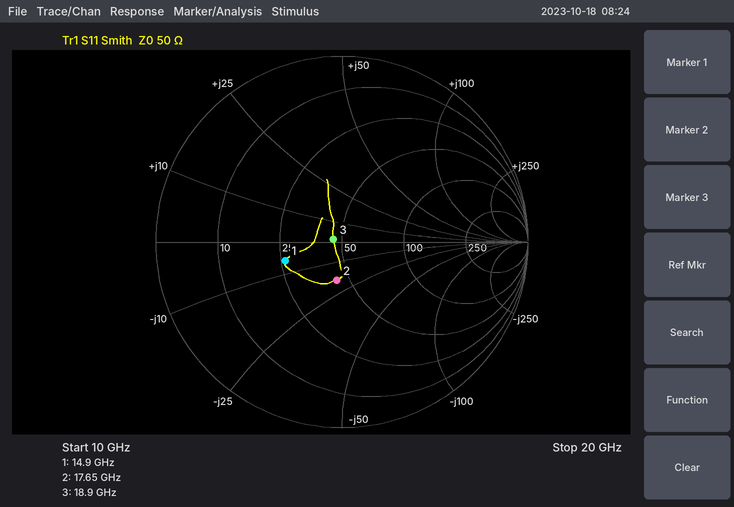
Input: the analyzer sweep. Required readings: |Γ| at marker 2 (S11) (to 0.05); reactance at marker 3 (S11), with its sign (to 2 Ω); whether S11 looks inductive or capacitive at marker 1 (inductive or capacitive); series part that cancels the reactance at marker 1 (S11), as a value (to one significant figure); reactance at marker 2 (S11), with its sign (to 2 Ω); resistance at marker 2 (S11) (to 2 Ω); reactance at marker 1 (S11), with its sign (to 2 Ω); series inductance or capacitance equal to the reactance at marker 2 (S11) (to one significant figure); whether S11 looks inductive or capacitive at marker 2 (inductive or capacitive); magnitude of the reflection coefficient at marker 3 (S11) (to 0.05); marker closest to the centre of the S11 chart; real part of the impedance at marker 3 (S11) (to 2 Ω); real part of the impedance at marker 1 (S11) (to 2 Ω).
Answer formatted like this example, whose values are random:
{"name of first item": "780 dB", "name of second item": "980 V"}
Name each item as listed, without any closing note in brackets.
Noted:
{"|Γ| at marker 2 (S11)": "0.20", "reactance at marker 3 (S11), with its sign": "+2 Ω", "whether S11 looks inductive or capacitive at marker 1": "capacitive", "series part that cancels the reactance at marker 1 (S11), as a value": "60 pH", "reactance at marker 2 (S11), with its sign": "-18 Ω", "resistance at marker 2 (S11)": "44 Ω", "reactance at marker 1 (S11), with its sign": "-6 Ω", "series inductance or capacitance equal to the reactance at marker 2 (S11)": "500 fF", "whether S11 looks inductive or capacitive at marker 2": "capacitive", "magnitude of the reflection coefficient at marker 3 (S11)": "0.05", "marker closest to the centre of the S11 chart": "marker 3", "real part of the impedance at marker 3 (S11)": "46 Ω", "real part of the impedance at marker 1 (S11)": "26 Ω"}
